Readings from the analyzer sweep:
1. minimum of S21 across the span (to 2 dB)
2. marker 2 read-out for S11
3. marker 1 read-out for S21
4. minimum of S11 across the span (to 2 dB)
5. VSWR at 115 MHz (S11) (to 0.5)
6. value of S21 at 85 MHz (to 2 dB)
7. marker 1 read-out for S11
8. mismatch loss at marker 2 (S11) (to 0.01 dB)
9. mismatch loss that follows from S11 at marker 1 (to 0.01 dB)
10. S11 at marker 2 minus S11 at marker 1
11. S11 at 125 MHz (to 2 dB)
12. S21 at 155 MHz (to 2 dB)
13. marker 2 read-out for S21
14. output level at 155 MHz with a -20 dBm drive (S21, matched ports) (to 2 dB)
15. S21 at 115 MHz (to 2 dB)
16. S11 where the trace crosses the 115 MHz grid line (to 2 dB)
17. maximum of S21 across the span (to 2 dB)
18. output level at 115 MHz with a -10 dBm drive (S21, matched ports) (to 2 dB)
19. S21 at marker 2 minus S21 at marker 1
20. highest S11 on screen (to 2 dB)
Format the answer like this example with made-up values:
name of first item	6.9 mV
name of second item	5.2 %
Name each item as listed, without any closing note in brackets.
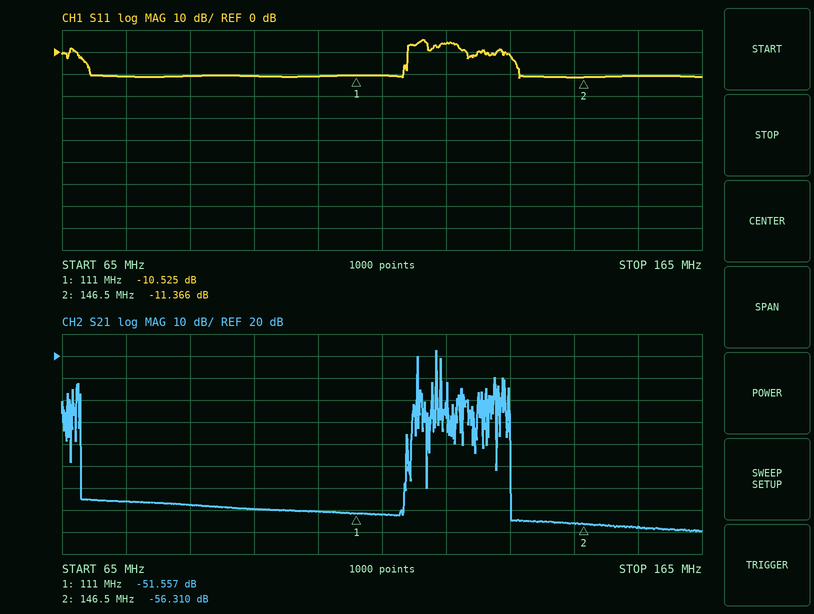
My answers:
minimum of S21 across the span	-60 dB
marker 2 read-out for S11	-11.366 dB
marker 1 read-out for S21	-51.557 dB
minimum of S11 across the span	-12 dB
VSWR at 115 MHz (S11)	2.0
value of S21 at 85 MHz	-48 dB
marker 1 read-out for S11	-10.525 dB
mismatch loss at marker 2 (S11)	0.33 dB
mismatch loss that follows from S11 at marker 1	0.40 dB
S11 at marker 2 minus S11 at marker 1	-0.841 dB
S11 at 125 MHz	4 dB
S21 at 155 MHz	-58 dB
marker 2 read-out for S21	-56.310 dB
output level at 155 MHz with a -20 dBm drive (S21, matched ports)	-78 dBm
S21 at 115 MHz	-52 dB
S11 where the trace crosses the 115 MHz grid line	-10 dB
maximum of S21 across the span	22 dB
output level at 115 MHz with a -10 dBm drive (S21, matched ports)	-62 dBm
S21 at marker 2 minus S21 at marker 1	-4.753 dB
highest S11 on screen	6 dB
